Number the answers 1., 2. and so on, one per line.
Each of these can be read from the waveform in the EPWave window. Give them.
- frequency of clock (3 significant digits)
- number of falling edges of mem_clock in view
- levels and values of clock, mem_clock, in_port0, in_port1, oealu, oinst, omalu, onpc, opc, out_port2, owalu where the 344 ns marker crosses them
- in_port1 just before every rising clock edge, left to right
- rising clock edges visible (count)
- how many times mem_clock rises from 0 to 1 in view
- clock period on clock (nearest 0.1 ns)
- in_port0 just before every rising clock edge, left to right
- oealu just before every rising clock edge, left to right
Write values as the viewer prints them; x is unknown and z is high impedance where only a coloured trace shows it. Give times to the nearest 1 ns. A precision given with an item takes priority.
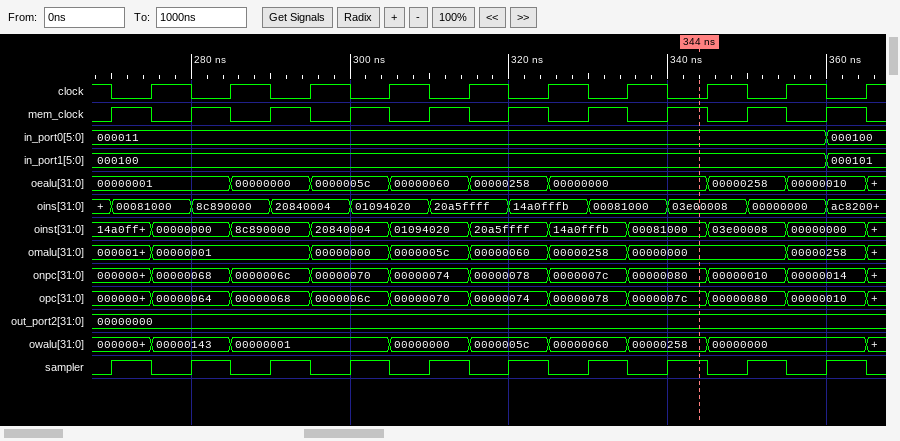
1. 100 MHz
2. 10
3. clock=0, mem_clock=1, in_port0=000011, in_port1=000100, oealu=00000000, oinst=00081000, omalu=00000000, onpc=00000080, opc=0000007c, out_port2=00000000, owalu=00000258
4. 000100, 000100, 000100, 000100, 000100, 000100, 000100, 000100, 000100, 000101
5. 10
6. 10
7. 10 ns
8. 000011, 000011, 000011, 000011, 000011, 000011, 000011, 000011, 000011, 000100
9. 00000001, 00000001, 00000000, 0000005c, 00000060, 00000258, 00000000, 00000000, 00000258, 00000010
